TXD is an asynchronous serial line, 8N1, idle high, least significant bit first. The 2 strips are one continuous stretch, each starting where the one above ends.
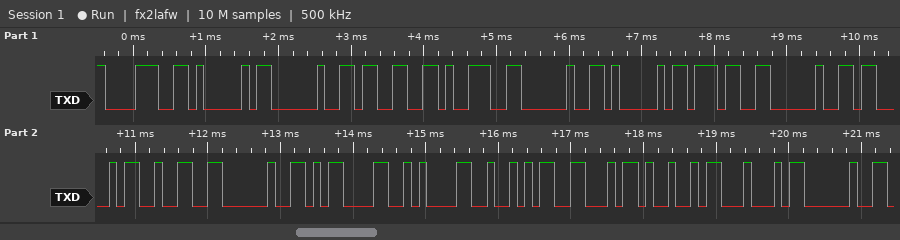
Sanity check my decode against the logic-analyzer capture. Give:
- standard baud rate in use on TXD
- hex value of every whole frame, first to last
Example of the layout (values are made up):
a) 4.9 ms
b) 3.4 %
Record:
a) 9600 baud
b) 0x38 0x41 0x20 0x33 0x39 0x20 0x41 0x37 0x20 0x43 0x32 0x20 0x0D 0x0A 0x52 0x46 0x49 0x44 0x20
